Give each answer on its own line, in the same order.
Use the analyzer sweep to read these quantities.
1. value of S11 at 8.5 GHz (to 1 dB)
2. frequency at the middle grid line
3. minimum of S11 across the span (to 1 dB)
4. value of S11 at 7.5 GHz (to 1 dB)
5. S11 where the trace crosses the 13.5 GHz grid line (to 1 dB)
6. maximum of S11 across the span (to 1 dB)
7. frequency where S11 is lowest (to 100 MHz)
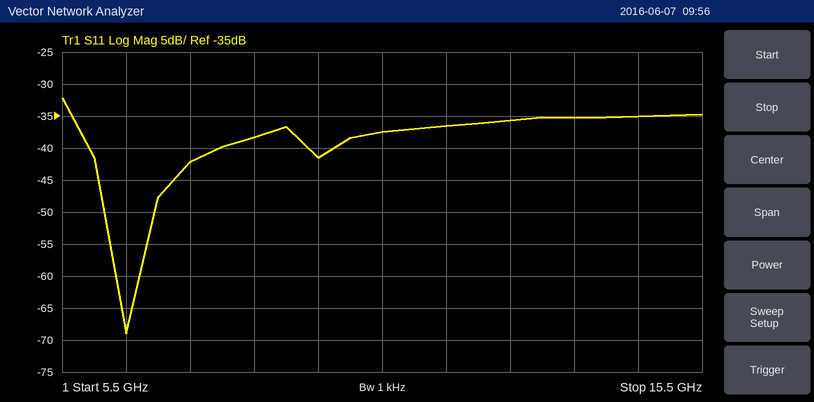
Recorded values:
-38 dB
10.5 GHz
-69 dB
-42 dB
-35 dB
-32 dB
6.5 GHz
